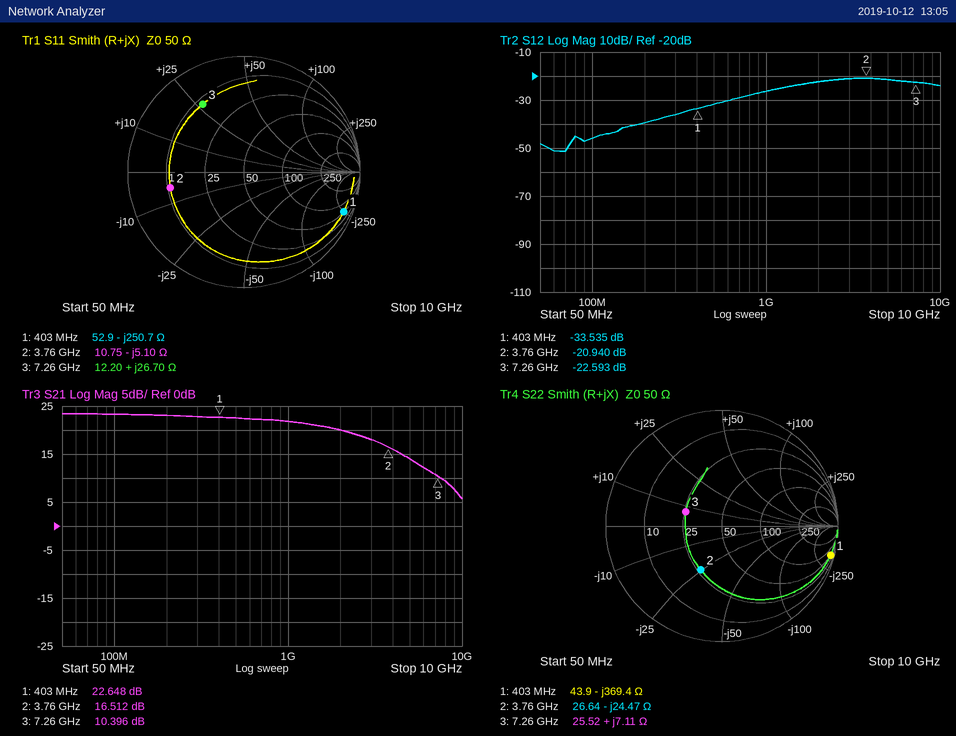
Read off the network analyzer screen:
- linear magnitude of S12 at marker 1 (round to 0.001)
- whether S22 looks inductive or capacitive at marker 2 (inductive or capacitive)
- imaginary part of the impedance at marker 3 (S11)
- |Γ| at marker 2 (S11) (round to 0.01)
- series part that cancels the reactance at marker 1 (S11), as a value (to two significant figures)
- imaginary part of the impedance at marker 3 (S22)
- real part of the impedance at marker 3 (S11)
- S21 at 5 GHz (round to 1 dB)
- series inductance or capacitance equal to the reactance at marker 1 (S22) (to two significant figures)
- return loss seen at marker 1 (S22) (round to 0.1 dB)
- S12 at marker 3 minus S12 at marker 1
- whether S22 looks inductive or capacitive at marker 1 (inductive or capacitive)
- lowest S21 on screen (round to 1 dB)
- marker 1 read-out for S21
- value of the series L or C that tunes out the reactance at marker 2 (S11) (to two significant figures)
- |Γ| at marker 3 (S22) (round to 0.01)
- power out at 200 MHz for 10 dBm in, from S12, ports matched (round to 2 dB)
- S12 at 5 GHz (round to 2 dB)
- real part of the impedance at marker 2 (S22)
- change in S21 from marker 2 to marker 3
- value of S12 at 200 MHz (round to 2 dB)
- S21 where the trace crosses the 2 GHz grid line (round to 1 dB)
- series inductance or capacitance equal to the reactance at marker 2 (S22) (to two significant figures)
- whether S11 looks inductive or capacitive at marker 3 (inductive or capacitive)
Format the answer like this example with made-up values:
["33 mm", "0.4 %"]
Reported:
["0.021", "capacitive", "+26.70 Ω", "0.65", "99 nH", "+7.11 Ω", "12.20 Ω", "14 dB", "1.1 pF", "0.3 dB", "10.942 dB", "capacitive", "6 dB", "22.648 dB", "220 pH", "0.34", "-30 dBm", "-22 dB", "26.64 Ω", "-6.116 dB", "-40 dB", "20 dB", "1.7 pF", "inductive"]
